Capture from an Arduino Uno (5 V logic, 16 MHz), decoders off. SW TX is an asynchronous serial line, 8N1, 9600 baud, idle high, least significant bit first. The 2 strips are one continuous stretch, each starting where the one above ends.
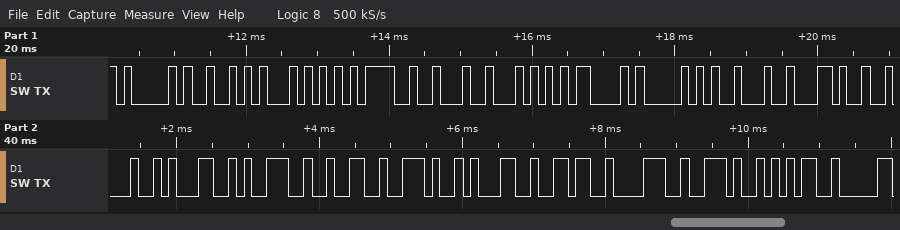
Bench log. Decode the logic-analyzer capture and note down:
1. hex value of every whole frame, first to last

41 52 54 3D 22 54 43 50 22 2C 22 31 39 32 2E 31 36 38 2E 35
